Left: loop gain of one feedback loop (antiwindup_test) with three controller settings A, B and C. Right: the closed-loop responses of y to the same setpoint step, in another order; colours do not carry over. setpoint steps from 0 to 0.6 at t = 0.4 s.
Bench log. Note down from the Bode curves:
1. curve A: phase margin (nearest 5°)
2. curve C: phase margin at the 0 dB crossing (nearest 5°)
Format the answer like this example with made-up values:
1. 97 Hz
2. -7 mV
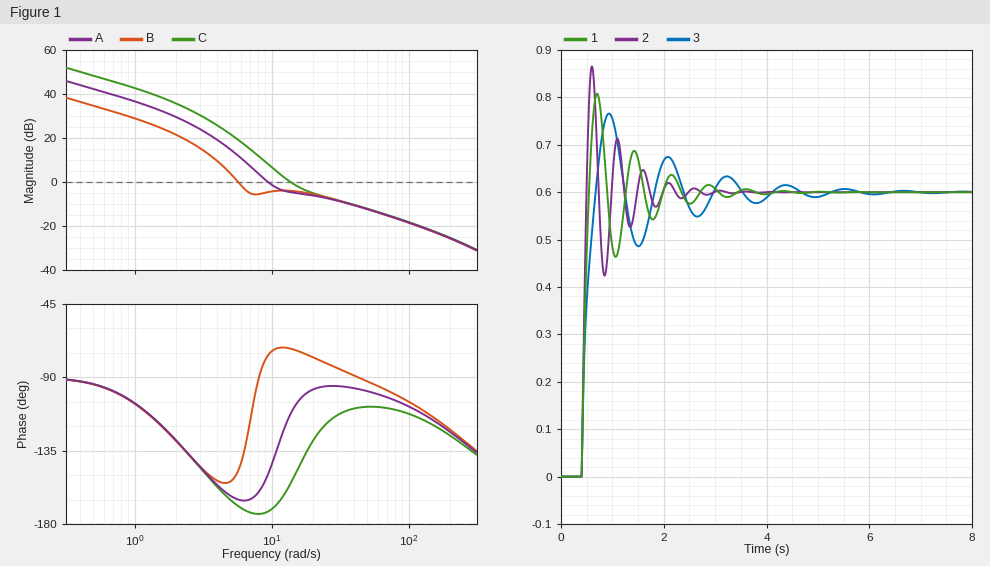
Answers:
1. 30°
2. 25°
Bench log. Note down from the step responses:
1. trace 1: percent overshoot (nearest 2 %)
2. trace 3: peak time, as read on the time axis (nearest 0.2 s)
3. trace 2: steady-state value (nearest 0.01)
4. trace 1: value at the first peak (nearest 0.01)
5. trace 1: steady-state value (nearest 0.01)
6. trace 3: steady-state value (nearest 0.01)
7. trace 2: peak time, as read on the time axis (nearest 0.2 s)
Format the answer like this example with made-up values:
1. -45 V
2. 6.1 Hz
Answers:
1. 34 %
2. 1.0 s
3. 0.60
4. 0.81
5. 0.60
6. 0.60
7. 0.6 s
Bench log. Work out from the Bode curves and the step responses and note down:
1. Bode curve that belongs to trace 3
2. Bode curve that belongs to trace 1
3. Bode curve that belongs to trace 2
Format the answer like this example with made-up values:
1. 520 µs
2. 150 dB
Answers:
1. B
2. A
3. C
